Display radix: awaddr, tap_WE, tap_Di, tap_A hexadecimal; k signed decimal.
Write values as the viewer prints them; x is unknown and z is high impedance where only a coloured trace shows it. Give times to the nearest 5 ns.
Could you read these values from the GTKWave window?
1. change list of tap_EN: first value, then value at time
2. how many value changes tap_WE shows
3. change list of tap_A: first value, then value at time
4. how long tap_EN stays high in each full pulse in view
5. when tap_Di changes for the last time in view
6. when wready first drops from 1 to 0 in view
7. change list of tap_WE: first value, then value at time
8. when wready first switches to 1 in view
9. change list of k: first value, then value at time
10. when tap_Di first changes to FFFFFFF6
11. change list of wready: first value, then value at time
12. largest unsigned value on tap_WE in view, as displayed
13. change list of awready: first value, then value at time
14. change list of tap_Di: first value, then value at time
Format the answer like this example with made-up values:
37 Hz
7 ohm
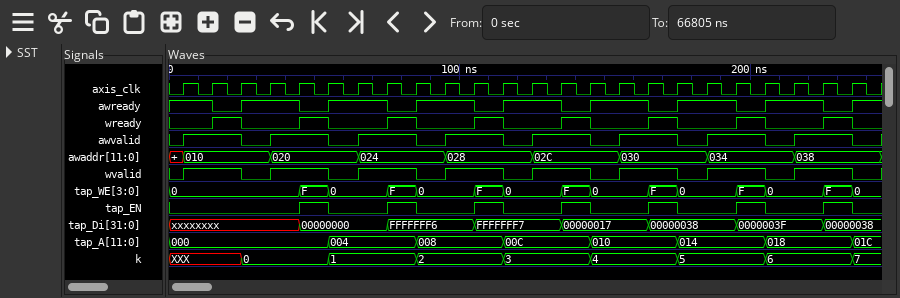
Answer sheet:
0, 1 at 45 ns, 0 at 55 ns, 1 at 75 ns, 0 at 85 ns, 1 at 105 ns, 0 at 115 ns, 1 at 135 ns, 0 at 145 ns, 1 at 165 ns, 0 at 175 ns, 1 at 195 ns, 0 at 205 ns, 1 at 225 ns, 0 at 235 ns
14
000, 004 at 55 ns, 008 at 85 ns, 00C at 115 ns, 010 at 145 ns, 014 at 175 ns, 018 at 205 ns, 01C at 235 ns
10 ns, 10 ns, 10 ns, 10 ns, 10 ns, 10 ns, 10 ns
225 ns
25 ns
0, F at 45 ns, 0 at 55 ns, F at 75 ns, 0 at 85 ns, F at 105 ns, 0 at 115 ns, F at 135 ns, 0 at 145 ns, F at 165 ns, 0 at 175 ns, F at 195 ns, 0 at 205 ns, F at 225 ns, 0 at 235 ns
15 ns
XXX, 0 at 25 ns, 1 at 55 ns, 2 at 85 ns, 3 at 115 ns, 4 at 145 ns, 5 at 175 ns, 6 at 205 ns, 7 at 235 ns
75 ns
0, 1 at 15 ns, 0 at 25 ns, 1 at 45 ns, 0 at 55 ns, 1 at 75 ns, 0 at 85 ns, 1 at 105 ns, 0 at 115 ns, 1 at 135 ns, 0 at 145 ns, 1 at 165 ns, 0 at 175 ns, 1 at 195 ns, 0 at 205 ns, 1 at 225 ns, 0 at 235 ns
F
1, 0 at 15 ns, 1 at 25 ns, 0 at 45 ns, 1 at 55 ns, 0 at 75 ns, 1 at 85 ns, 0 at 105 ns, 1 at 115 ns, 0 at 135 ns, 1 at 145 ns, 0 at 165 ns, 1 at 175 ns, 0 at 195 ns, 1 at 205 ns, 0 at 225 ns, 1 at 235 ns
xxxxxxxx, 00000000 at 45 ns, FFFFFFF6 at 75 ns, FFFFFFF7 at 105 ns, 00000017 at 135 ns, 00000038 at 165 ns, 0000003F at 195 ns, 00000038 at 225 ns
